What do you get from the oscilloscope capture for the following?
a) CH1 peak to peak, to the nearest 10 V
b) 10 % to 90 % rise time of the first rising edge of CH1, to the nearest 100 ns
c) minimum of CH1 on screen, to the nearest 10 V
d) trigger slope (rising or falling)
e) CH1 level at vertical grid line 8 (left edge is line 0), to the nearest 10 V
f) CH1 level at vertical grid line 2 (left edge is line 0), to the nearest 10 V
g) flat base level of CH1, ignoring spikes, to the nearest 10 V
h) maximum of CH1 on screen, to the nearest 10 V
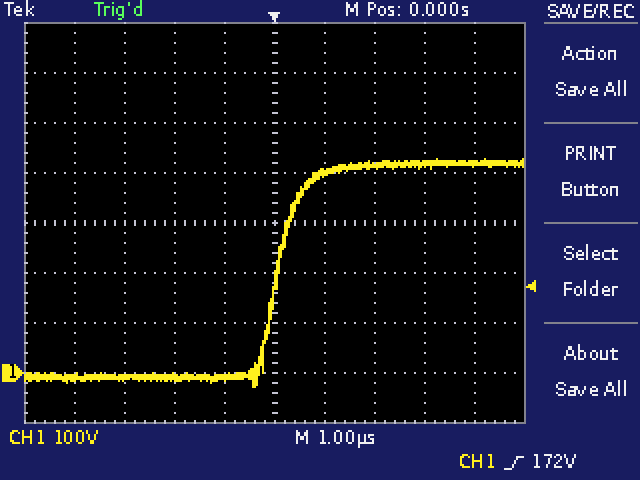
460 V
900 ns
-30 V
rising
420 V
-10 V
-10 V
430 V
